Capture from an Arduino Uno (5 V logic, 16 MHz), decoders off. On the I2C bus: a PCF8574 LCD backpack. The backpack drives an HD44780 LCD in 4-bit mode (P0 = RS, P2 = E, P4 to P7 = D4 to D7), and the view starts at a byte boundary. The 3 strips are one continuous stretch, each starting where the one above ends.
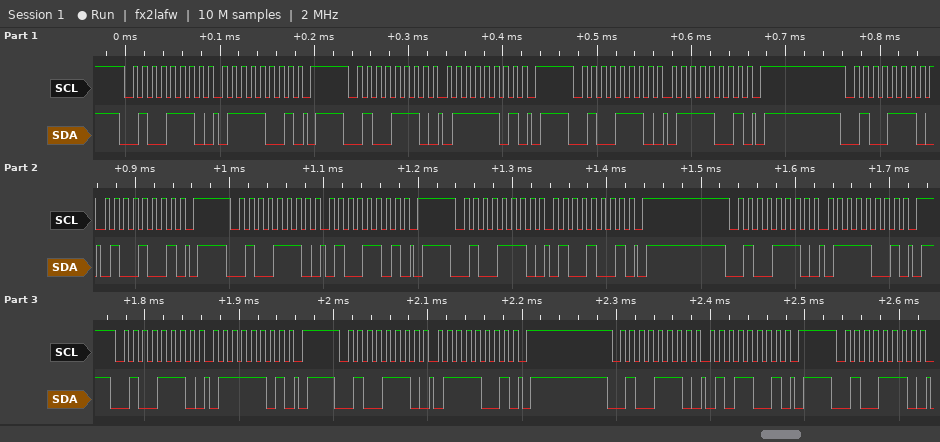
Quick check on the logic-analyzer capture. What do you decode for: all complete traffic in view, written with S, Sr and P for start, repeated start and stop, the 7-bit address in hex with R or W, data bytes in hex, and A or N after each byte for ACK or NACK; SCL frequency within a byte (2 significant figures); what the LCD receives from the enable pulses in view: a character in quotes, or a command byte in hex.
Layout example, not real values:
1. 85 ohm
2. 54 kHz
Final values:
1. S 27W A 79 A P S 27W A 7D A P S 27W A 79 A P S 27W A 49 A P S 27W A 4D A P S 27W A 49 A P S 27W A 79 A P S 27W A 7D A P S 27W A 79 A P S 27W A 59 A P S 27W A
2. 100 kHz
3. 't'
